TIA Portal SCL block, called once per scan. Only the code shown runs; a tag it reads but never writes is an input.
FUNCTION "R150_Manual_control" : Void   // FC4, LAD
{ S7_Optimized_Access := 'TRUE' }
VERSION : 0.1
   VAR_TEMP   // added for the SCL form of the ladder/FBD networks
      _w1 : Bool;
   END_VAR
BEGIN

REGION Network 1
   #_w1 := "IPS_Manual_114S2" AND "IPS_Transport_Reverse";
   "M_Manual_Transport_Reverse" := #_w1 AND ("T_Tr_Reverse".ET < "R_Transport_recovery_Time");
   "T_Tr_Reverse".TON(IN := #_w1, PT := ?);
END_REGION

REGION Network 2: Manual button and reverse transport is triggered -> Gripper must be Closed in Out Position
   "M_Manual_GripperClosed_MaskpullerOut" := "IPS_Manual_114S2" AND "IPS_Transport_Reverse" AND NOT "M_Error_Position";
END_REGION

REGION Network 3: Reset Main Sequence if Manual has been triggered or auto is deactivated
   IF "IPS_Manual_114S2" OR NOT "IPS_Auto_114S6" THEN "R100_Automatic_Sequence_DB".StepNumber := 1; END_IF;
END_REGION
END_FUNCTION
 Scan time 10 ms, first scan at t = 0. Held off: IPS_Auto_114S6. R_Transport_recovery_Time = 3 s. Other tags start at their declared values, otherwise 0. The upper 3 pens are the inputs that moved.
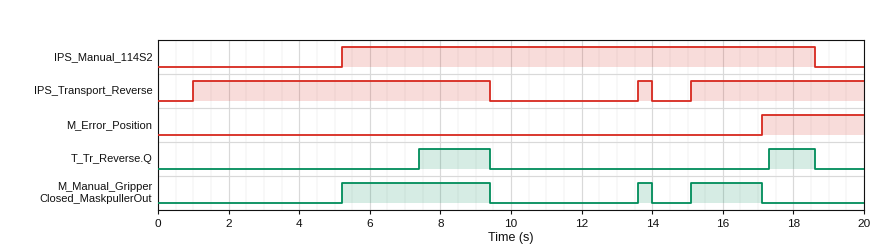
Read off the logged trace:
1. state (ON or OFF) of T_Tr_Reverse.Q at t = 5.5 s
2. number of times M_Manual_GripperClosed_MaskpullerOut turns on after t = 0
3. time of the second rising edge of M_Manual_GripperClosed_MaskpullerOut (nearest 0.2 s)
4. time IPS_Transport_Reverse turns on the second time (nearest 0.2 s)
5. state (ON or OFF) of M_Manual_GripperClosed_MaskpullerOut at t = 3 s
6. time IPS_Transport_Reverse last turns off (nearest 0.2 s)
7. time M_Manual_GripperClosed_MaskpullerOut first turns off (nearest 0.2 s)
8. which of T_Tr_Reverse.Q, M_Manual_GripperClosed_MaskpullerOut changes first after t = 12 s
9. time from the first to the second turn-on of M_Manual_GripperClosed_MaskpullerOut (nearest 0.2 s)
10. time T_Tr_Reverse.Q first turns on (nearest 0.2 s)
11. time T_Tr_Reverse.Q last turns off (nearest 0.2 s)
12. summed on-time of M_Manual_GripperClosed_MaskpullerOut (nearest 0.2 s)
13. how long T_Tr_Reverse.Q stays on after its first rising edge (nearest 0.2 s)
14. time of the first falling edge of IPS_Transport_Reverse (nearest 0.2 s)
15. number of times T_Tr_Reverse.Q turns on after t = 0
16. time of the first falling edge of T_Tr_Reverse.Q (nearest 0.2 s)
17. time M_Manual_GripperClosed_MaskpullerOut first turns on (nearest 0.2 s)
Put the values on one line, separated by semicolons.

OFF; 3; 13.6 s; 13.6 s; OFF; 14.0 s; 9.4 s; M_Manual_GripperClosed_MaskpullerOut; 8.4 s; 7.4 s; 18.6 s; 6.6 s; 2.0 s; 9.4 s; 2; 9.4 s; 5.2 s
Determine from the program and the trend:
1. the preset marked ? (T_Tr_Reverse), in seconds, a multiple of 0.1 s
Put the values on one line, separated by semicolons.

2.2 s
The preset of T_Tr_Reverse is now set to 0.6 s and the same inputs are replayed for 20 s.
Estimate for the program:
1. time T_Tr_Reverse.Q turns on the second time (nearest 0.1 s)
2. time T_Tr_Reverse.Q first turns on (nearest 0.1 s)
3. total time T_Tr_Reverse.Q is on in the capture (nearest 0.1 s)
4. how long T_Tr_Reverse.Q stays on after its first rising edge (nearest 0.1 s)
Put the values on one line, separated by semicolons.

15.7 s; 5.8 s; 6.5 s; 3.6 s
